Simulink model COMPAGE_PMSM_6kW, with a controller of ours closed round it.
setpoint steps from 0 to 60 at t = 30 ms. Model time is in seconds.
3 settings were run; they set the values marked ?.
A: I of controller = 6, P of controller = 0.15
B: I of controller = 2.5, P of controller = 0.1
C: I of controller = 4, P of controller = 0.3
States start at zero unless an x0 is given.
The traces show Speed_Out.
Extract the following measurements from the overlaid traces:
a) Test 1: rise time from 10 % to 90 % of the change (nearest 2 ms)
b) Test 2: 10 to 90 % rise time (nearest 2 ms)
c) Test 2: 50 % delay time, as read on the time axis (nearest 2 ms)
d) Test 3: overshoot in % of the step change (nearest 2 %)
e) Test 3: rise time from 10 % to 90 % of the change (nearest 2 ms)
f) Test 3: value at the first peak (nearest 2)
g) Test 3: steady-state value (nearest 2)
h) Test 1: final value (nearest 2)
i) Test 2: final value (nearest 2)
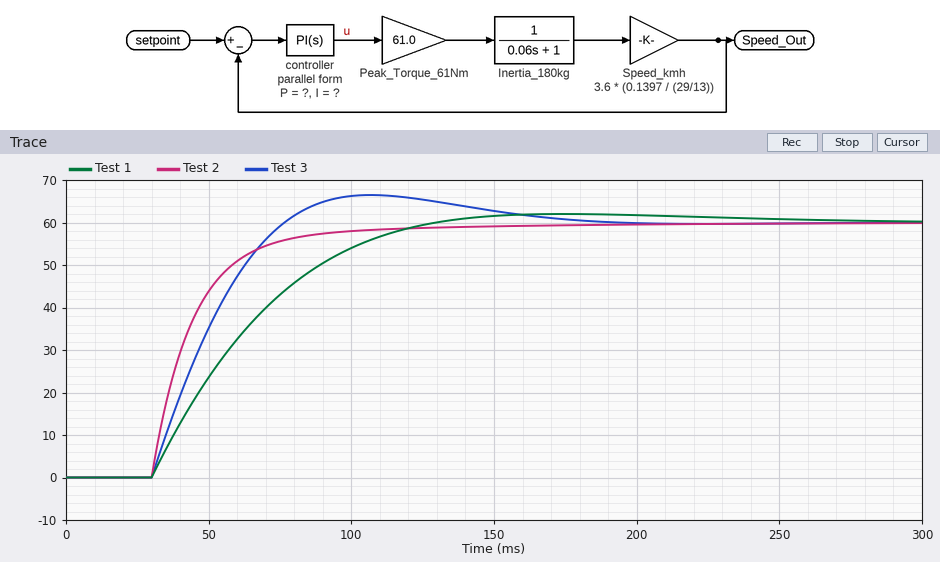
66 ms
36 ms
40 ms
10 %
34 ms
66
60
60
60
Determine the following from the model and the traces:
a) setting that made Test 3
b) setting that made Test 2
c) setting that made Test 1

A
C
B
